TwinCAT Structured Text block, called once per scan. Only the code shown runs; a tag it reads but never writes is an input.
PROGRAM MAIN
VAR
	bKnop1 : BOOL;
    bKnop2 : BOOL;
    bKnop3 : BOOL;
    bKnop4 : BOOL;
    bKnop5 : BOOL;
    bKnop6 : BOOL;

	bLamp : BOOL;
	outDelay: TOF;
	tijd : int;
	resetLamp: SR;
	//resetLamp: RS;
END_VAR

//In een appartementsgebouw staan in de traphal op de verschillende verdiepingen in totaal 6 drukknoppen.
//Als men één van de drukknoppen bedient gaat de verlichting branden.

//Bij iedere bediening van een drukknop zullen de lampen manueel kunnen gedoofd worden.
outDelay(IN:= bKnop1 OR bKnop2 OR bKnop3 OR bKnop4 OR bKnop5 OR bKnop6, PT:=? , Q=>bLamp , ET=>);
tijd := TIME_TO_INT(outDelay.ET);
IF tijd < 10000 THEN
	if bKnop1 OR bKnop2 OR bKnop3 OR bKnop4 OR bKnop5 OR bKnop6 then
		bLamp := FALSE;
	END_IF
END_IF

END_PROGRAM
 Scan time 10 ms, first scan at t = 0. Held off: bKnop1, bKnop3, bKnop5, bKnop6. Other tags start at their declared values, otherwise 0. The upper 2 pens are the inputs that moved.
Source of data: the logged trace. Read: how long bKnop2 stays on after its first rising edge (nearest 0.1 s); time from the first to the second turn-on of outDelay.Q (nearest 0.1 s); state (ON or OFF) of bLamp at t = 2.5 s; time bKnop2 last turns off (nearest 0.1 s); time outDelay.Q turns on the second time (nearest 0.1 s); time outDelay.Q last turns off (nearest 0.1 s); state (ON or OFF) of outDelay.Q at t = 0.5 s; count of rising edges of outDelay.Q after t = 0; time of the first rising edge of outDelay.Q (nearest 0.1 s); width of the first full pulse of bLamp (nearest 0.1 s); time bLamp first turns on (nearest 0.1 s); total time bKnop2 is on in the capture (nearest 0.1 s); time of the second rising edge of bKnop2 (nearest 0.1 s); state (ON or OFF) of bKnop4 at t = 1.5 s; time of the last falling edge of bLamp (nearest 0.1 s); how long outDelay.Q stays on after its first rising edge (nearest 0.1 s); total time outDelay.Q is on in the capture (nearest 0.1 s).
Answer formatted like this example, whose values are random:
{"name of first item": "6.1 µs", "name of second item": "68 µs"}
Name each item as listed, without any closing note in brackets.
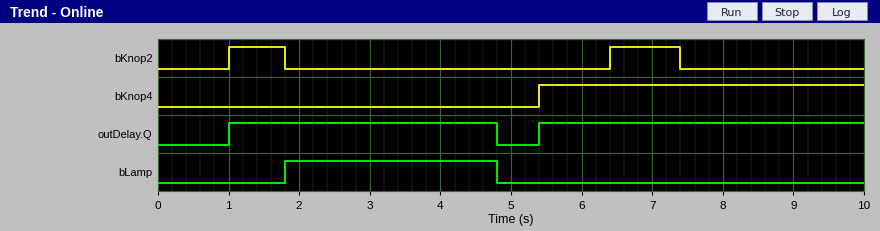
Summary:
{"how long bKnop2 stays on after its first rising edge": "0.8 s", "time from the first to the second turn-on of outDelay.Q": "4.4 s", "state (ON or OFF) of bLamp at t = 2.5 s": "ON", "time bKnop2 last turns off": "7.4 s", "time outDelay.Q turns on the second time": "5.4 s", "time outDelay.Q last turns off": "4.8 s", "state (ON or OFF) of outDelay.Q at t = 0.5 s": "OFF", "count of rising edges of outDelay.Q after t = 0": "2", "time of the first rising edge of outDelay.Q": "1.0 s", "width of the first full pulse of bLamp": "3.0 s", "time bLamp first turns on": "1.8 s", "total time bKnop2 is on in the capture": "1.8 s", "time of the second rising edge of bKnop2": "6.4 s", "state (ON or OFF) of bKnop4 at t = 1.5 s": "OFF", "time of the last falling edge of bLamp": "4.8 s", "how long outDelay.Q stays on after its first rising edge": "3.8 s", "total time outDelay.Q is on in the capture": "8.4 s"}
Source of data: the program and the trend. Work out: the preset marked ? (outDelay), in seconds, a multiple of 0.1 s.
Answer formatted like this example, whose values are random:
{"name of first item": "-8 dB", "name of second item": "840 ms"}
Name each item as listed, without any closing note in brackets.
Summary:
{"the preset marked ? (outDelay), in seconds, a multiple of 0.1 s": "3.0 s"}
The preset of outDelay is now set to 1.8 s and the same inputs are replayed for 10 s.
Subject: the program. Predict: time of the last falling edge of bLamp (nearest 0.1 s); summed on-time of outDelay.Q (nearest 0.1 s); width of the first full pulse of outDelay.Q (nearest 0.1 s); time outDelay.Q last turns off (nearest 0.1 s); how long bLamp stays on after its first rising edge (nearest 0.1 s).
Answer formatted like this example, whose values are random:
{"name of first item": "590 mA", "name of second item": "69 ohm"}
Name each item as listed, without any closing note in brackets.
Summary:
{"time of the last falling edge of bLamp": "3.6 s", "summed on-time of outDelay.Q": "7.2 s", "width of the first full pulse of outDelay.Q": "2.6 s", "time outDelay.Q last turns off": "3.6 s", "how long bLamp stays on after its first rising edge": "1.8 s"}
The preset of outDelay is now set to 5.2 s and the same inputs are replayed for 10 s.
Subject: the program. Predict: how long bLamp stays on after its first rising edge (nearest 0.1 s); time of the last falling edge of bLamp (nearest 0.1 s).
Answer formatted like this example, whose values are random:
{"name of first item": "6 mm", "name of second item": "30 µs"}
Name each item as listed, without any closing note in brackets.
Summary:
{"how long bLamp stays on after its first rising edge": "3.6 s", "time of the last falling edge of bLamp": "5.4 s"}
